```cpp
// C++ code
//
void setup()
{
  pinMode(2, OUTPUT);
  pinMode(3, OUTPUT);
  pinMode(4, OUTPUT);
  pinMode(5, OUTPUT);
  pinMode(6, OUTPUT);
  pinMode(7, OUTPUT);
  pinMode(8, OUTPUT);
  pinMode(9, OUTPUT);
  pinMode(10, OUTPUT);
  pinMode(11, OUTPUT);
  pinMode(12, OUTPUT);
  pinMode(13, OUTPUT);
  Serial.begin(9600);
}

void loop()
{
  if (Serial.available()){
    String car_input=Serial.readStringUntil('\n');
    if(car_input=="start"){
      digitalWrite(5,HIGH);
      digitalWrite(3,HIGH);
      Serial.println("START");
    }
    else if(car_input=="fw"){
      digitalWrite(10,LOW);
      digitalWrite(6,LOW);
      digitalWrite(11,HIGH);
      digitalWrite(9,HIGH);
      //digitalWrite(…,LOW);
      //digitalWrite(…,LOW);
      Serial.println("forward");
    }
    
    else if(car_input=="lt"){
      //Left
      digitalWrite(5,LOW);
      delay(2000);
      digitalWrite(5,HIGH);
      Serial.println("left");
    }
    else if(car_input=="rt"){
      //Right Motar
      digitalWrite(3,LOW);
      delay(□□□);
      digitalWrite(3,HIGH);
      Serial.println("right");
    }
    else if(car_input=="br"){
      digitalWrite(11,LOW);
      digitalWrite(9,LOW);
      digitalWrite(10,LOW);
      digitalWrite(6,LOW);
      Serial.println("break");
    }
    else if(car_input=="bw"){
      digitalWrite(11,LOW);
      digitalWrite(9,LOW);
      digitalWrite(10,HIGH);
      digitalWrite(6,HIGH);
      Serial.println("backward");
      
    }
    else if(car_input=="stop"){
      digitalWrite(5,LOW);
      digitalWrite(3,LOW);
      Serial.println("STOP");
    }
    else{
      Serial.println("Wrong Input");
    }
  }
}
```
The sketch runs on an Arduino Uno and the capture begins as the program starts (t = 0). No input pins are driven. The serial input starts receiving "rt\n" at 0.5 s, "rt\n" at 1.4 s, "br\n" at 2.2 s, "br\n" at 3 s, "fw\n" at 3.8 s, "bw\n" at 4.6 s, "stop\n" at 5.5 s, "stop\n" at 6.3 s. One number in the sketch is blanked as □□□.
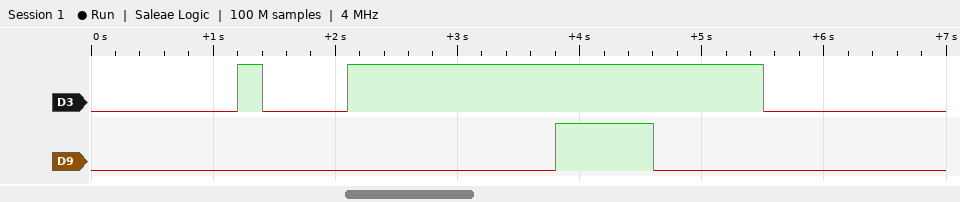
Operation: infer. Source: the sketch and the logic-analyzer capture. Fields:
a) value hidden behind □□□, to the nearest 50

700
